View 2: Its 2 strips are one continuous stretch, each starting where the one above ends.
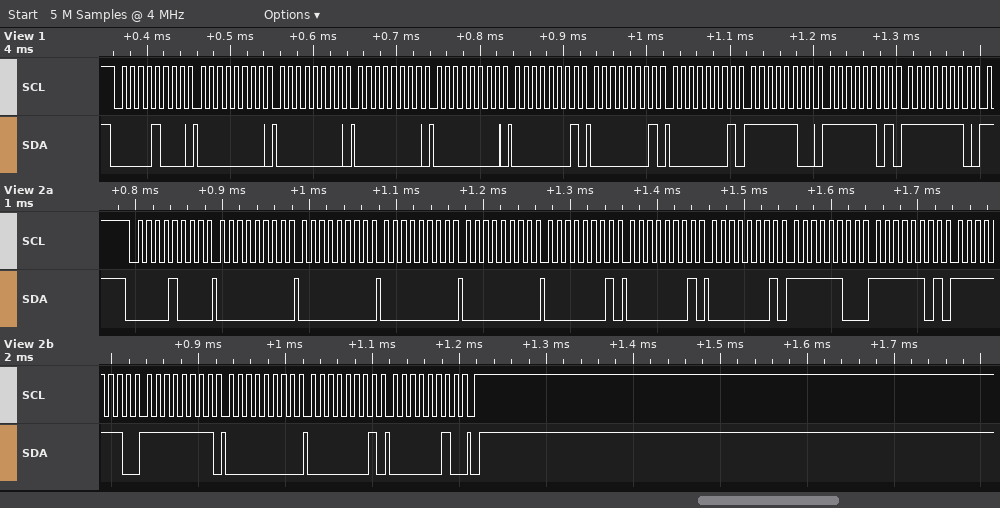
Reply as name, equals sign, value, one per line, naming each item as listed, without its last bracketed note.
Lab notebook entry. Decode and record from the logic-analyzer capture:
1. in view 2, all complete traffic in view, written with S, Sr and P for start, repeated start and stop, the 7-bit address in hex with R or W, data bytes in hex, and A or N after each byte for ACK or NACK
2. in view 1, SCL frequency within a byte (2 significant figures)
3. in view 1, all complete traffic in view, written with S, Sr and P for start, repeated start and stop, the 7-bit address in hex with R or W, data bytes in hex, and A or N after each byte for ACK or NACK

in view 2, all complete traffic in view, written with S, Sr and P for start, repeated start and stop, the 7-bit address in hex with R or W, data bytes in hex, and A or N after each byte for ACK or NACK = S 04W A 00 A 00 A 00 A 00 A 01 A 01 A 01 A FC A FD A FE A FF A 00 A 01 A 02 A P
in view 1, SCL frequency within a byte = 100 kHz
in view 1, all complete traffic in view, written with S, Sr and P for start, repeated start and stop, the 7-bit address in hex with R or W, data bytes in hex, and A or N after each byte for ACK or NACK = S 04W A 00 A 00 A 00 A 00 A 01 A 01 A 01 A FC A FD A FE A
